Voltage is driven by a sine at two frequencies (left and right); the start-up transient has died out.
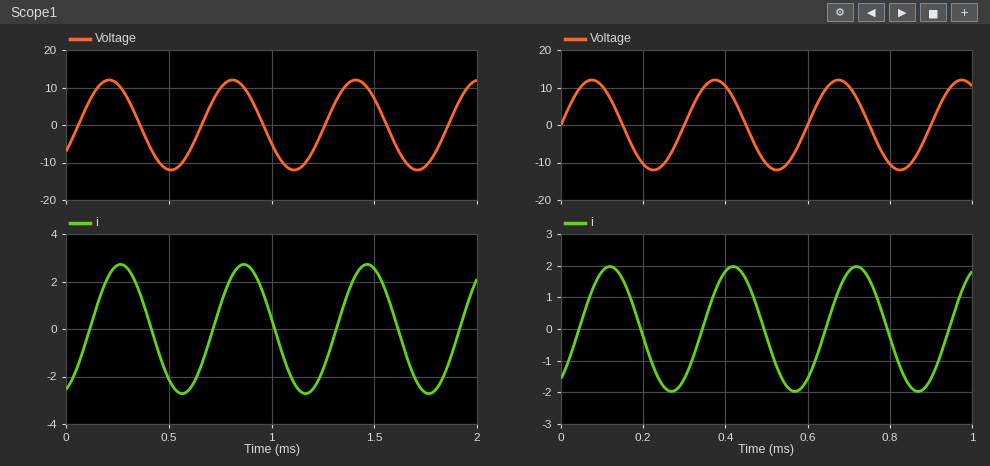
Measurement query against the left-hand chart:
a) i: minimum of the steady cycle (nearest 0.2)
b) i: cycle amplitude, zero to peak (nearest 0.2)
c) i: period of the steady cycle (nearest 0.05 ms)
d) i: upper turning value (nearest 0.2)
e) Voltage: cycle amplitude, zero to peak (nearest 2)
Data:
-2.8
2.8
0.60 ms
2.8
12
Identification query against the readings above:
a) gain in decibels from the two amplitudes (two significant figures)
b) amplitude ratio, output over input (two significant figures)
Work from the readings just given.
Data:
-13 dB
0.23
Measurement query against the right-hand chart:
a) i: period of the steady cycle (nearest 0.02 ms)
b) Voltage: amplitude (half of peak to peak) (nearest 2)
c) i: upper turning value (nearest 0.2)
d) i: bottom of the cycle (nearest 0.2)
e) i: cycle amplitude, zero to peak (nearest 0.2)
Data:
0.30 ms
12
2.0
-2.0
2.0
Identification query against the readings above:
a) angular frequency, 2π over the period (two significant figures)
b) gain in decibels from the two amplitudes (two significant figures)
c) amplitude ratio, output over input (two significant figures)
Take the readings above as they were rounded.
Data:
21 rad/ms
-16 dB
0.17
